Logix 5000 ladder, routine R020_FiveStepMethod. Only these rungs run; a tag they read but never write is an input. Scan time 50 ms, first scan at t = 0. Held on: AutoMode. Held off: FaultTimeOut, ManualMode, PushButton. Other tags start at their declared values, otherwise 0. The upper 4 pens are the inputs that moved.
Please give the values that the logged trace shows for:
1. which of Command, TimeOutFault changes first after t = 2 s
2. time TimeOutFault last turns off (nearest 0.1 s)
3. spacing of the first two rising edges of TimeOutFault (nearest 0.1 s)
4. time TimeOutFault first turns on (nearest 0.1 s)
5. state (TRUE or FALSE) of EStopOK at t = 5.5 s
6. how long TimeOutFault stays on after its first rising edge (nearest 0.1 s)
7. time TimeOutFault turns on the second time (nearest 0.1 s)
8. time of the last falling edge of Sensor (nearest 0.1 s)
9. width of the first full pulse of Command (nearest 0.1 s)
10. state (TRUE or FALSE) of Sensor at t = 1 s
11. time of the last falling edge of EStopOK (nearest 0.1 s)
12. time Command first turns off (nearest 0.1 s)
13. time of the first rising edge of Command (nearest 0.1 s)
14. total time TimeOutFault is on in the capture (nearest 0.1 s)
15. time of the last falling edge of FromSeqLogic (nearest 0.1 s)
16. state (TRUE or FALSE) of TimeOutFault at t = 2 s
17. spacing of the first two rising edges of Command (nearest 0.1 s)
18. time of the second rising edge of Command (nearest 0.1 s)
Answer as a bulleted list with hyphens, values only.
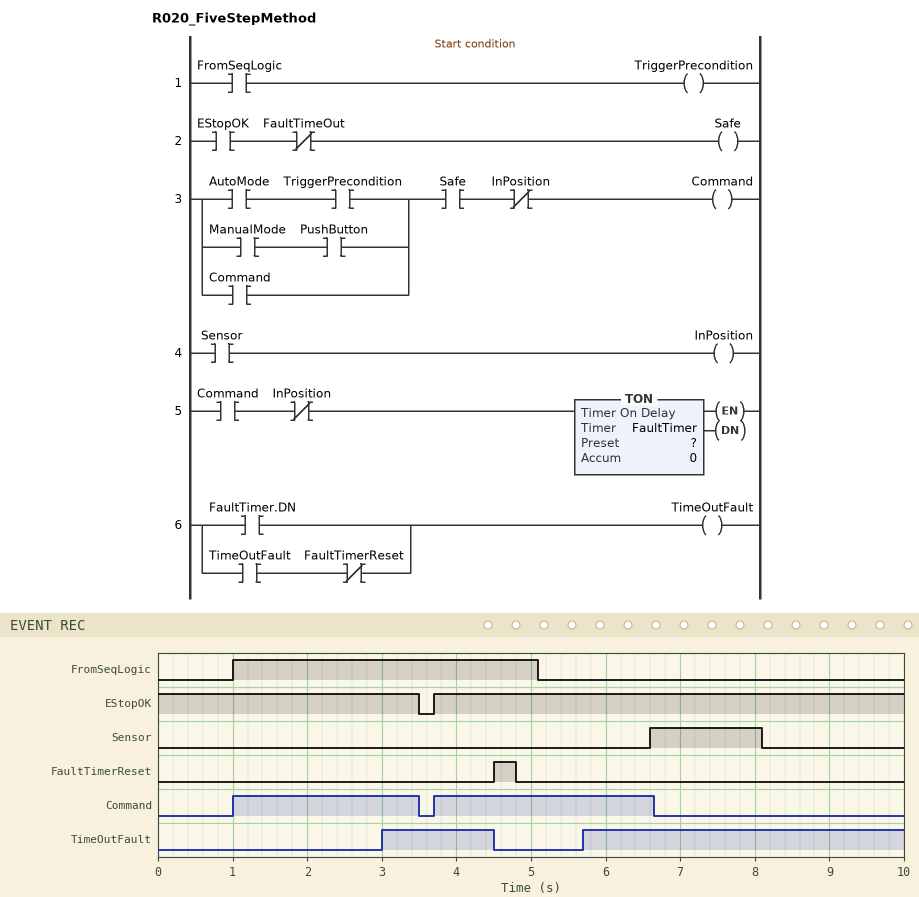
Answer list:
- TimeOutFault
- 4.5 s
- 2.7 s
- 3.0 s
- TRUE
- 1.5 s
- 5.7 s
- 8.1 s
- 2.5 s
- FALSE
- 3.5 s
- 3.5 s
- 1.0 s
- 5.8 s
- 5.1 s
- FALSE
- 2.7 s
- 3.7 s
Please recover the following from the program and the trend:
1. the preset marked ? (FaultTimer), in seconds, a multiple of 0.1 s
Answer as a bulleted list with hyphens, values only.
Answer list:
- 2.0 s
